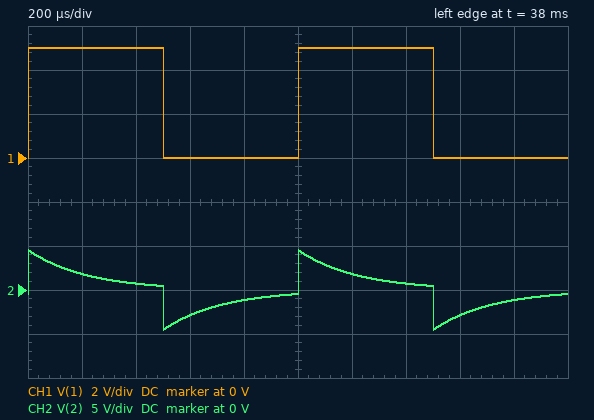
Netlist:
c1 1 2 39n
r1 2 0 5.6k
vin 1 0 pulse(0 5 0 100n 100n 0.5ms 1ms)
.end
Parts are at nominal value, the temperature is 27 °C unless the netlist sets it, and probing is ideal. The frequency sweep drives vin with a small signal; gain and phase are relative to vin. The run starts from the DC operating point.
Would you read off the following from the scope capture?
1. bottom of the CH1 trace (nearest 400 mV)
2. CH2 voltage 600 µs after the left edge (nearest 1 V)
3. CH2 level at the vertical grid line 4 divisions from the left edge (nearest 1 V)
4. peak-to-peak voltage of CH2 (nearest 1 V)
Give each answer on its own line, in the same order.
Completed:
0 V
-3 V
-1 V
9 V
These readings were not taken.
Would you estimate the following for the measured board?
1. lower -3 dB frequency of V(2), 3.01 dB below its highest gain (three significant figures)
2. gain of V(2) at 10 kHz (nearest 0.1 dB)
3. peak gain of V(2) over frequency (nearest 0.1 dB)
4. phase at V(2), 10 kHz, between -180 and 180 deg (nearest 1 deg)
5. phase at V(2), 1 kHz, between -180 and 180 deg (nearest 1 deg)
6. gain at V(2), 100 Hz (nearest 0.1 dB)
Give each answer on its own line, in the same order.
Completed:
729 Hz
0 dB
0 dB
4 deg
36 deg
-17.3 dB
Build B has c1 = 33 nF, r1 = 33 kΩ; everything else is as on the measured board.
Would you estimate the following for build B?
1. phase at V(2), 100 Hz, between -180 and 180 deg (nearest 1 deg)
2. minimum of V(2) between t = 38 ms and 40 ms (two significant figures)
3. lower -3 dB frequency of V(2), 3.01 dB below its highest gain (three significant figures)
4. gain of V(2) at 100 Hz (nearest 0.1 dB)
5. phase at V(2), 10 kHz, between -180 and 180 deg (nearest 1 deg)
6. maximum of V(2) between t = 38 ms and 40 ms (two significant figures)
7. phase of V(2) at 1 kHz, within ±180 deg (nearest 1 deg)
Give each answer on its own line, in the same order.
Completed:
56 deg
-3.1 V
146 Hz
-5.0 dB
1 deg
3.1 V
8 deg
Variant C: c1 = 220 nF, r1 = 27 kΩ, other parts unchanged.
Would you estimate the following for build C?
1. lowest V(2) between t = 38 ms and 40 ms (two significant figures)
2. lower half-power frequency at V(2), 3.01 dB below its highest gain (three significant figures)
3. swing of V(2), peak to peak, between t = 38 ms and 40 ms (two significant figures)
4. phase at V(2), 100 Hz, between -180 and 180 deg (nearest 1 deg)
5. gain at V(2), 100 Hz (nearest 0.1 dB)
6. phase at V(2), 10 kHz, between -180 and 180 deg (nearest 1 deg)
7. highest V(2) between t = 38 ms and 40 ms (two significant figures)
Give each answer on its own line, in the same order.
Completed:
-2.6 V
26.8 Hz
5.2 V
15 deg
-0.3 dB
0 deg
2.6 V
